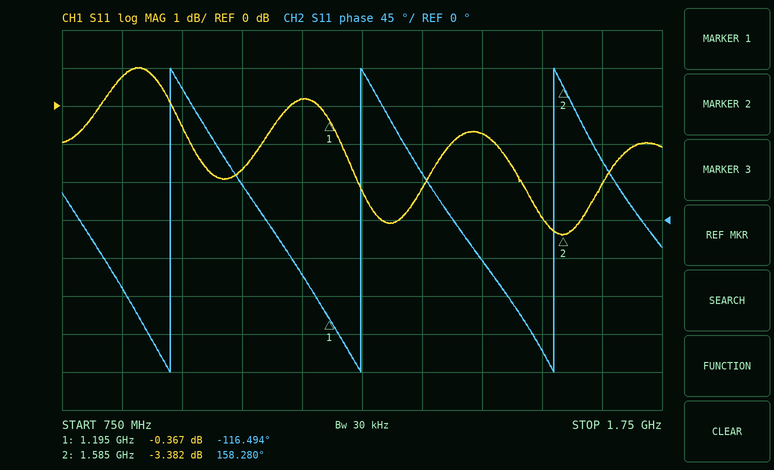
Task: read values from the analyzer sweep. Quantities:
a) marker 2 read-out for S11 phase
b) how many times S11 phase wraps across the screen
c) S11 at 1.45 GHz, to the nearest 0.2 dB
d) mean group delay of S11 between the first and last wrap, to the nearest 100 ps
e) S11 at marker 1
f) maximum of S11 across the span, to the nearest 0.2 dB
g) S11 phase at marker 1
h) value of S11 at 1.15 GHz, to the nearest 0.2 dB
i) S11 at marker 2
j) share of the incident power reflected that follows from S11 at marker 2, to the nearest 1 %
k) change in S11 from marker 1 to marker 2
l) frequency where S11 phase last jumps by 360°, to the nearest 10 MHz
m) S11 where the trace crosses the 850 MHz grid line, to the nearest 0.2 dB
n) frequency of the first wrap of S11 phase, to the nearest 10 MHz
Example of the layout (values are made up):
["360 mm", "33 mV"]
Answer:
["158.280°", "3", "-0.8 dB", "3.1 ns", "-0.367 dB", "1.0 dB", "-116.494°", "0.2 dB", "-3.382 dB", "46 %", "-3.015 dB", "1.57 GHz", "0.8 dB", "930 MHz"]
